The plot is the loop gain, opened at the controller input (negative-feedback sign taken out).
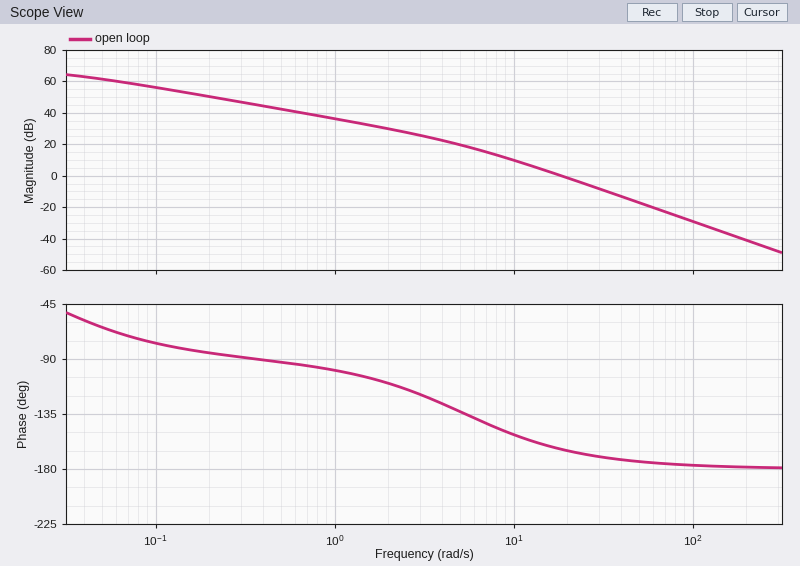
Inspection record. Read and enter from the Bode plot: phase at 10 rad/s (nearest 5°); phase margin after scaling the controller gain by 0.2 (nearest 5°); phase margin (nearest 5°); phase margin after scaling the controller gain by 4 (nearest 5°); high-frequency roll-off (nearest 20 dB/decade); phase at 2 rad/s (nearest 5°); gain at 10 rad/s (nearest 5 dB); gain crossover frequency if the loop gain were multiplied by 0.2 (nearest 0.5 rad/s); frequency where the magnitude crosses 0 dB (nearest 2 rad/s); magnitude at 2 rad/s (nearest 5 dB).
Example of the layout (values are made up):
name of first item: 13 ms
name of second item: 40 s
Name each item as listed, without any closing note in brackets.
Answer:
phase at 10 rad/s: -150°
phase margin after scaling the controller gain by 0.2: 35°
phase margin: 15°
phase margin after scaling the controller gain by 4: 10°
high-frequency roll-off: -40 dB/decade
phase at 2 rad/s: -110°
gain at 10 rad/s: 10 dB
gain crossover frequency if the loop gain were multiplied by 0.2: 7.5 rad/s
frequency where the magnitude crosses 0 dB: 18 rad/s
magnitude at 2 rad/s: 30 dB
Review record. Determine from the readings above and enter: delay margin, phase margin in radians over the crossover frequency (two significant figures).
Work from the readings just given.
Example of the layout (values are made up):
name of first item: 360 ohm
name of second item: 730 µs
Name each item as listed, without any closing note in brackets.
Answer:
delay margin, phase margin in radians over the crossover frequency: 0.015 s
